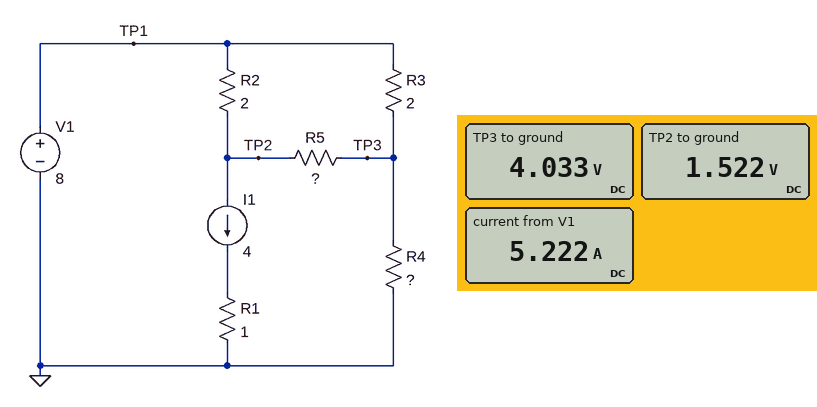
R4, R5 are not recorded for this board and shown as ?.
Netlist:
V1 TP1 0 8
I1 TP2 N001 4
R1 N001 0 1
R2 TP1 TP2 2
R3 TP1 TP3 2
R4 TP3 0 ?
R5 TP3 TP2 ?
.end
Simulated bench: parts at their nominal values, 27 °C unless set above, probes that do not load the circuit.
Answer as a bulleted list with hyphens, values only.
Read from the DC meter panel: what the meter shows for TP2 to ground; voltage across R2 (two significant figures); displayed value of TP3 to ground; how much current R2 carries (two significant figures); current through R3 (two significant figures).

- 1.522 V
- 6.5 V
- 4.033 V
- 3.2 A
- 2.0 A
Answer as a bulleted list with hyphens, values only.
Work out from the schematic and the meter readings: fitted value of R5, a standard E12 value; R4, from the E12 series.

- 3.3 Ω
- 3.3 Ω
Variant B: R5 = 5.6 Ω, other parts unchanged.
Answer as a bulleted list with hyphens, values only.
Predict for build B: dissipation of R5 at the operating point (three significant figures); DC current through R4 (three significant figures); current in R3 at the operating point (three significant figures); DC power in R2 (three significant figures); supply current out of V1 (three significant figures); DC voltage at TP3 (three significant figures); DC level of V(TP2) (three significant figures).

- 1.78 W
- 1.30 A
- 1.86 A
- 23.6 W
- 5.30 A
- 4.28 V
- 1.13 V
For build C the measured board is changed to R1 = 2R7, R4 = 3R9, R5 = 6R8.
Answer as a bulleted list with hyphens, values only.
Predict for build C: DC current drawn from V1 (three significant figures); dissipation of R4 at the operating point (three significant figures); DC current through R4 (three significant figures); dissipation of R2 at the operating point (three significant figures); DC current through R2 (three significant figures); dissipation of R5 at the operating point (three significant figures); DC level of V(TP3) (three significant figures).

- 5.18 A
- 5.42 W
- 1.18 A
- 24.2 W
- 3.48 A
- 1.86 W
- 4.60 V
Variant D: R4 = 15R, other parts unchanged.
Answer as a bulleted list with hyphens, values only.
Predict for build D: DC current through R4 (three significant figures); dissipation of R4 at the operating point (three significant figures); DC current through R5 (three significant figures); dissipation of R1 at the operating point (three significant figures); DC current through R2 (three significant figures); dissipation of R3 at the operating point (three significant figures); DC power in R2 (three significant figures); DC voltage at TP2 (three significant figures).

- 353 mA
- 1.87 W
- 999 mA
- 16.0 W
- 3.00 A
- 3.66 W
- 18.0 W
- 2.00 V
